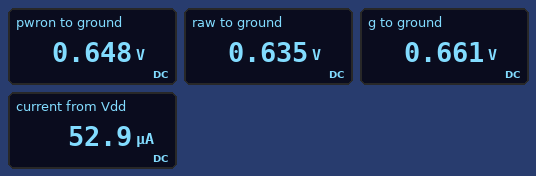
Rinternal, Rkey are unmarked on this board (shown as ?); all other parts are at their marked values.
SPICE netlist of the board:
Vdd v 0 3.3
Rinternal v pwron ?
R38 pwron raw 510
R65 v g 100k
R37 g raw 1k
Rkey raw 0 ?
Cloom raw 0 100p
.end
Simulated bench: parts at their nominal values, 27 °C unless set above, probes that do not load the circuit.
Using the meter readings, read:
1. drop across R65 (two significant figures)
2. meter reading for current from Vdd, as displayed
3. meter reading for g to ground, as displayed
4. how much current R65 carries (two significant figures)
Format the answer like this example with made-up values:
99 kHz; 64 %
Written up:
2.6 V; 52.9 µA; 0.661 V; 26 µA
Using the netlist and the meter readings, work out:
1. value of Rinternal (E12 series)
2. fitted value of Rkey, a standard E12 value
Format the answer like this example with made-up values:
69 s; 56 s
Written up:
100 kΩ; 12 kΩ
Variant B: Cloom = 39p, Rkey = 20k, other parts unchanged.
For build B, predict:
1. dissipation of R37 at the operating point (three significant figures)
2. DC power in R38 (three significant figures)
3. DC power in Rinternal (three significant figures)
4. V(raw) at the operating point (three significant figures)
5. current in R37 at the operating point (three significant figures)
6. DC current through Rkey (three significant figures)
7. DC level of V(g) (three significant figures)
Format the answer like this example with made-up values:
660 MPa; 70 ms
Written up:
547 nW; 282 nW; 55.2 µW; 938 mV; 23.4 µA; 46.9 µA; 961 mV
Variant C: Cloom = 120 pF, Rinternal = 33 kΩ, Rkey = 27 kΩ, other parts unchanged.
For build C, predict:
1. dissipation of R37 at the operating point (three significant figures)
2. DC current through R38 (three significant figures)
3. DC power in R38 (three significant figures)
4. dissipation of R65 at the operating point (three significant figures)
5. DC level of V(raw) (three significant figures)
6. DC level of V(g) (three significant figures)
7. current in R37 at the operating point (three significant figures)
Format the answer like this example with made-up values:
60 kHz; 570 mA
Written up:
248 nW; 47.5 µA; 1.15 µW; 24.8 µW; 1.71 V; 1.72 V; 15.8 µA
